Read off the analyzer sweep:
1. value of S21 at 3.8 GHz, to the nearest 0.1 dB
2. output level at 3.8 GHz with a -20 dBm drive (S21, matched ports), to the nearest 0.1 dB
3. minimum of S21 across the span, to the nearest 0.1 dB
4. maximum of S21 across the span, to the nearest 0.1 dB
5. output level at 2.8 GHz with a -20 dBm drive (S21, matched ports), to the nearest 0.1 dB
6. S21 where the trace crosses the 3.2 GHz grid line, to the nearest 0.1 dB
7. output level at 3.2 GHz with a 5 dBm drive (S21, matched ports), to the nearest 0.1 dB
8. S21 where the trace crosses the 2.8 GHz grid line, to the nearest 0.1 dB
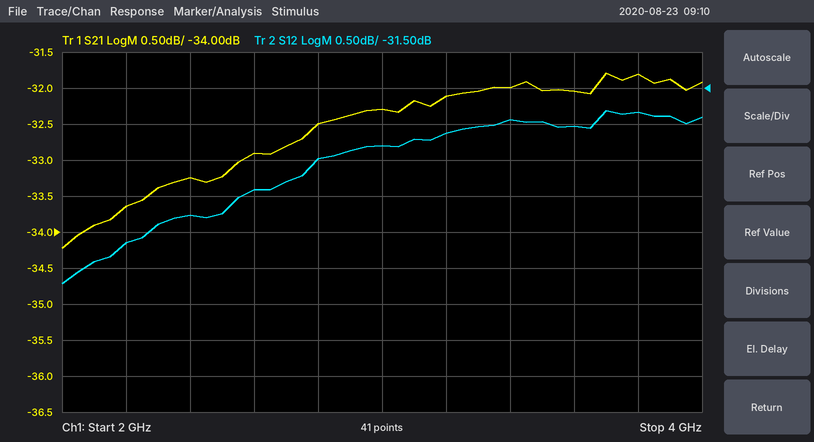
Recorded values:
-31.8 dB
-51.8 dBm
-34.2 dB
-31.8 dB
-52.5 dBm
-32.1 dB
-27.1 dBm
-32.5 dB
